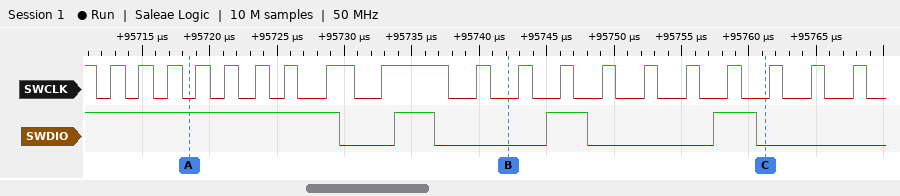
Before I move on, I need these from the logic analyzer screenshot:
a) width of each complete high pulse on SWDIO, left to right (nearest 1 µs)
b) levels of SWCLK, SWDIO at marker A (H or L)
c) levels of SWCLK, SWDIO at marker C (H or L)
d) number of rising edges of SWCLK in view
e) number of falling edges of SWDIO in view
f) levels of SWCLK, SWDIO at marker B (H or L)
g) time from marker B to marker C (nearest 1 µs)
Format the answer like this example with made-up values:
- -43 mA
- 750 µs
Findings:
- 3 µs, 3 µs, 3 µs
- SWCLK=L, SWDIO=H
- SWCLK=L, SWDIO=L
- 19
- 4
- SWCLK=L, SWDIO=L
- 19 µs
